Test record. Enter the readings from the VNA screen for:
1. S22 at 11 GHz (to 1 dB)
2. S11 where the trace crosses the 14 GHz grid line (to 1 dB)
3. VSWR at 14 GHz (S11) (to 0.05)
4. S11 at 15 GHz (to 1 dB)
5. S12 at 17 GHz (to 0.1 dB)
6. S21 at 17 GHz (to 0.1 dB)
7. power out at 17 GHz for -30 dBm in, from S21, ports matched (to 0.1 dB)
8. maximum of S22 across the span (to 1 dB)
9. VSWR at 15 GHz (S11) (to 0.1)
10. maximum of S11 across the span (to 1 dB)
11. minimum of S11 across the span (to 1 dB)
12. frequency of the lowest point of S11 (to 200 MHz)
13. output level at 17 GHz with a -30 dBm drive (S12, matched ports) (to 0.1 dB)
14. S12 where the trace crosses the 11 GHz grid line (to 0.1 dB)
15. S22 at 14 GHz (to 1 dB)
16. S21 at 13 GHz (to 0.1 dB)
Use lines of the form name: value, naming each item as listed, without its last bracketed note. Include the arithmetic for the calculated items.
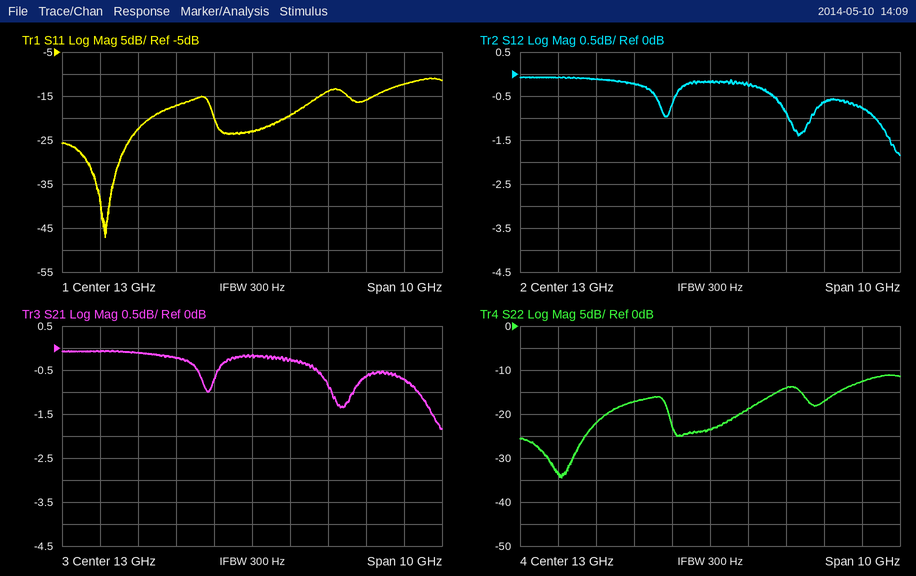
S22 at 11 GHz: -17 dB
S11 where the trace crosses the 14 GHz grid line: -19 dB
VSWR at 14 GHz (S11): |Γ| = 10^(-19/20) = 0.1122; VSWR = (1 + 0.1122)/(1 − 0.1122) ≈ 1.25
S11 at 15 GHz: -14 dB
S12 at 17 GHz: -0.8 dB
S21 at 17 GHz: -0.7 dB
power out at 17 GHz for -30 dBm in, from S21, ports matched: -30 dBm + (-0.7 dB) = -30.7 dBm
maximum of S22 across the span: -11 dB
VSWR at 15 GHz (S11): |Γ| = 10^(-14/20) = 0.1995; VSWR = (1 + 0.1995)/(1 − 0.1995) ≈ 1.5
maximum of S11 across the span: -11 dB
minimum of S11 across the span: -47 dB
frequency of the lowest point of S11: 9.2 GHz
output level at 17 GHz with a -30 dBm drive (S12, matched ports): -30 dBm + (-0.8 dB) = -30.8 dBm
S12 where the trace crosses the 11 GHz grid line: -0.2 dB
S22 at 14 GHz: -19 dB
S21 at 13 GHz: -0.2 dB
